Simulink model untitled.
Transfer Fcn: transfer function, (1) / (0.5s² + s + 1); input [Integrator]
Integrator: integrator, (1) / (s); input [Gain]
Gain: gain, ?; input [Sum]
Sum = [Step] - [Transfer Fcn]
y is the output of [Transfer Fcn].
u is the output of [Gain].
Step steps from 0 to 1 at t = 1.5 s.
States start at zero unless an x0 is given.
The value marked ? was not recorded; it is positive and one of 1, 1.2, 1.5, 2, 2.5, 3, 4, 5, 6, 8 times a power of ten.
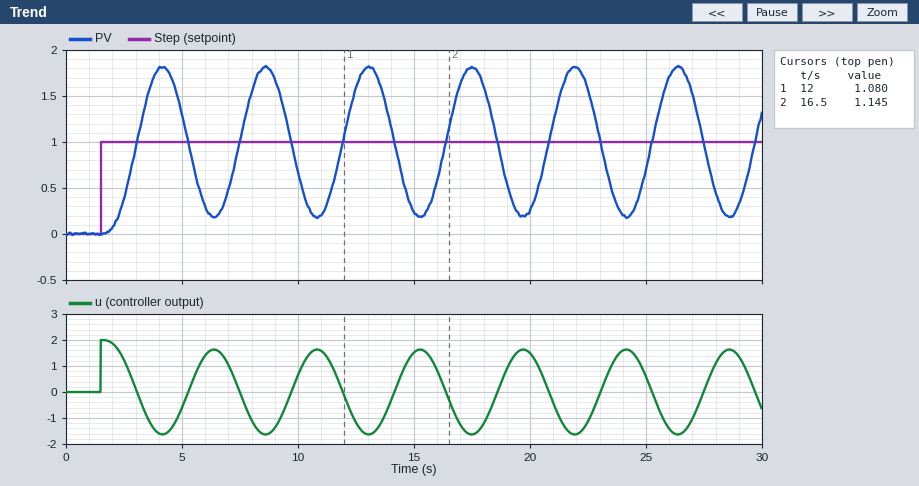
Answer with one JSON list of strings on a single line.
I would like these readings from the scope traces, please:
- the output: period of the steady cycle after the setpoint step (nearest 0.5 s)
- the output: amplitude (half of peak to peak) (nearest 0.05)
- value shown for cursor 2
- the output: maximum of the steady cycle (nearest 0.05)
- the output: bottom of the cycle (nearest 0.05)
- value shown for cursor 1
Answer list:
["4.5 s", "0.80", "1.145", "1.80", "0.20", "1.080"]
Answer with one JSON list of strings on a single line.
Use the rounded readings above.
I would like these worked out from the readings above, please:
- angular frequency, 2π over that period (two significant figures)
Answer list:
["1.4 rad/s"]
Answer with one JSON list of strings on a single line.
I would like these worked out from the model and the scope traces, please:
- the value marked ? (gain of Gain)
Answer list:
["2"]
